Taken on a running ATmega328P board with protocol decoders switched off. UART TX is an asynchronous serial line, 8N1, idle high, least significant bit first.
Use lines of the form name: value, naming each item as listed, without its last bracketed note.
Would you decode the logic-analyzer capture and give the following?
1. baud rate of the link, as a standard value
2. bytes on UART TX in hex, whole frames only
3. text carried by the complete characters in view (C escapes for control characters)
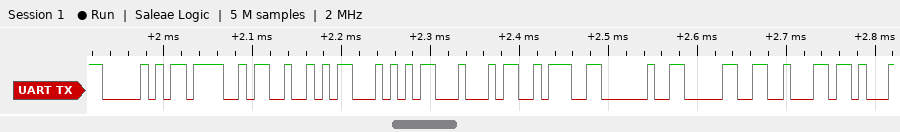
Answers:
baud rate of the link, as a standard value: 115200 baud
bytes on UART TX in hex, whole frames only: 0x50 0x4F 0x52 0x54 0x44 0x3A 0x20 0x30 0x62
text carried by the complete characters in view: "PORTD: 0b"
